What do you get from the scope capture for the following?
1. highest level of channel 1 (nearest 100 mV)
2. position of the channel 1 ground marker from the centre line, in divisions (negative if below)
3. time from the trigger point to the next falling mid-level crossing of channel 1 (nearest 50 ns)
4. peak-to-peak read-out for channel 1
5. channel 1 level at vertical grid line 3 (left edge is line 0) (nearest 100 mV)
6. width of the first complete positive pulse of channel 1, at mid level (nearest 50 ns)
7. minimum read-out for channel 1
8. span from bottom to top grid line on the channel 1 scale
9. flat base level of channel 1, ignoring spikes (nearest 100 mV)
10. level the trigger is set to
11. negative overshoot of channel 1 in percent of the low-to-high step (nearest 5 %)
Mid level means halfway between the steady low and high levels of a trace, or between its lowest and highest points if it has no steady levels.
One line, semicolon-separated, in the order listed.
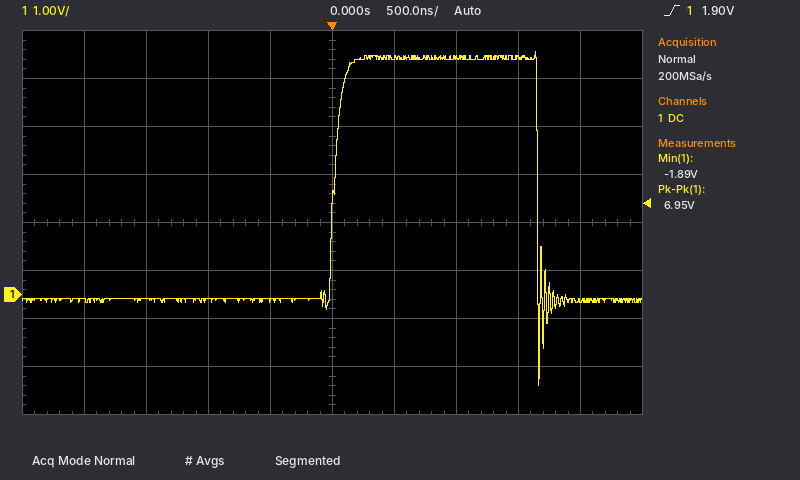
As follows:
5.1 V; -1.5 div; 1.65 µs; 6.95 V; -100 mV; 1.65 µs; -1.89 V; 8 V; -100 mV; 1.90 V; 35 %
